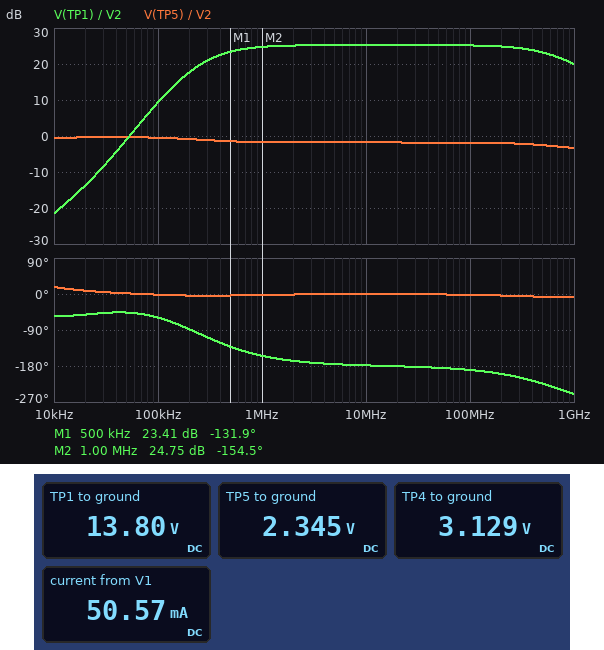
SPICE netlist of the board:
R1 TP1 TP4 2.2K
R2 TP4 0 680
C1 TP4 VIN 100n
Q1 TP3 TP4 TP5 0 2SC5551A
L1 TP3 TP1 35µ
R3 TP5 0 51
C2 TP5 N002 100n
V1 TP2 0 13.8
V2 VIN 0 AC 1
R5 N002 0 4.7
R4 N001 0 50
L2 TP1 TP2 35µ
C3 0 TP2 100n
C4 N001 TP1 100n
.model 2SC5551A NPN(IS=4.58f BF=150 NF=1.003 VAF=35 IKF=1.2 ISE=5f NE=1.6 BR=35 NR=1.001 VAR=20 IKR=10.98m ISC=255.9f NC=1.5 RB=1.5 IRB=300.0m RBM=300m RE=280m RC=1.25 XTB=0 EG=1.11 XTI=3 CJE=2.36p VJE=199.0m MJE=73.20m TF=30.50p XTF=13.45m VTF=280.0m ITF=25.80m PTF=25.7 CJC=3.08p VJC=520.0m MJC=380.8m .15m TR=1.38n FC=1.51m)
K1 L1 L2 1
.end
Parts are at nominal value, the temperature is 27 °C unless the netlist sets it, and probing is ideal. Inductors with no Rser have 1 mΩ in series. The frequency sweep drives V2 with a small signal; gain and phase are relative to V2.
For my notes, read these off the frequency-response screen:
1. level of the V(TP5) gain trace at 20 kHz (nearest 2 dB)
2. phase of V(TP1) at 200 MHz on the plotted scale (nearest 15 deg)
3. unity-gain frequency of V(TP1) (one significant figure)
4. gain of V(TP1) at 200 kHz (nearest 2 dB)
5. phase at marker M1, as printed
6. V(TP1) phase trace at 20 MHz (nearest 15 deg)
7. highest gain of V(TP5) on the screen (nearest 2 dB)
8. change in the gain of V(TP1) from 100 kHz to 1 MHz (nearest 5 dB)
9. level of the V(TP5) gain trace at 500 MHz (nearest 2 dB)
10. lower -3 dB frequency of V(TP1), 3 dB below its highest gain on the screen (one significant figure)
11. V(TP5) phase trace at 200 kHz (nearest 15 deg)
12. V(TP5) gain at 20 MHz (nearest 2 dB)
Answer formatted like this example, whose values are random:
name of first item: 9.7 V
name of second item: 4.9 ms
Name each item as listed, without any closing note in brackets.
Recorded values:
level of the V(TP5) gain trace at 20 kHz: 0 dB
phase of V(TP1) at 200 MHz on the plotted scale: -195 deg
unity-gain frequency of V(TP1): 50 kHz
gain of V(TP1) at 200 kHz: 18 dB
phase at marker M1, as printed: -131.9 deg
V(TP1) phase trace at 20 MHz: -180 deg
highest gain of V(TP5) on the screen: 0 dB
change in the gain of V(TP1) from 100 kHz to 1 MHz: 15 dB
level of the V(TP5) gain trace at 500 MHz: -2 dB
lower -3 dB frequency of V(TP1), 3 dB below its highest gain on the screen: 400 kHz
V(TP5) phase trace at 200 kHz: 0 deg
V(TP5) gain at 20 MHz: -2 dB
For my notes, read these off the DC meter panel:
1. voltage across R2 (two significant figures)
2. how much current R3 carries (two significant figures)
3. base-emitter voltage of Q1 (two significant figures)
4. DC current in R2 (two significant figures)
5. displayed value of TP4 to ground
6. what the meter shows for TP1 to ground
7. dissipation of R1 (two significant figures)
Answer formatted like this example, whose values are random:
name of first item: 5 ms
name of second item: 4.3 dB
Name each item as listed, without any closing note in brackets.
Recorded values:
voltage across R2: 3.1 V
how much current R3 carries: 46 mA
base-emitter voltage of Q1: 780 mV
DC current in R2: 4.6 mA
displayed value of TP4 to ground: 3.129 V
what the meter shows for TP1 to ground: 13.80 V
dissipation of R1: 52 mW
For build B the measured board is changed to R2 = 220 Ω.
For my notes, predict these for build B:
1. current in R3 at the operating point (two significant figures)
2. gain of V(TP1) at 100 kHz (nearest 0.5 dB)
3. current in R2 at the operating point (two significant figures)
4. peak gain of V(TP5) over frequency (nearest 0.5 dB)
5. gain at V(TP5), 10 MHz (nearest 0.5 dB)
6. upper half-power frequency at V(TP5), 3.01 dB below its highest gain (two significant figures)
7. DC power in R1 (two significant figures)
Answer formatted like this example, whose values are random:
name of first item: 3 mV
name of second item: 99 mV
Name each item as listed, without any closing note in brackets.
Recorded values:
current in R3 at the operating point: 10 mA
gain of V(TP1) at 100 kHz: 8.5 dB
current in R2 at the operating point: 5.7 mA
peak gain of V(TP5) over frequency: -1.0 dB
gain at V(TP5), 10 MHz: -4.5 dB
upper half-power frequency at V(TP5), 3.01 dB below its highest gain: 540 kHz
DC power in R1: 72 mW
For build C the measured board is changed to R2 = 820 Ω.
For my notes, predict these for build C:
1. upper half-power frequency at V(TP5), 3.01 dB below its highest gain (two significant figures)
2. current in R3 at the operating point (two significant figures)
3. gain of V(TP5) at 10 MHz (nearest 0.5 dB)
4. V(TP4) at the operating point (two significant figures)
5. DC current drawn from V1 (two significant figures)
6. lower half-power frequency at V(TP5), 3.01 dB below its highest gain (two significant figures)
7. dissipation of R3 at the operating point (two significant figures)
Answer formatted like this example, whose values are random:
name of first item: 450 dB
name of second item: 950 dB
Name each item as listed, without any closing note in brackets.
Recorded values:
upper half-power frequency at V(TP5), 3.01 dB below its highest gain: 1.1 GHz
current in R3 at the operating point: 54 mA
gain of V(TP5) at 10 MHz: -1.5 dB
V(TP4) at the operating point: 3.6 V
DC current drawn from V1: 59 mA
lower half-power frequency at V(TP5), 3.01 dB below its highest gain: 2.8 kHz
dissipation of R3 at the operating point: 150 mW
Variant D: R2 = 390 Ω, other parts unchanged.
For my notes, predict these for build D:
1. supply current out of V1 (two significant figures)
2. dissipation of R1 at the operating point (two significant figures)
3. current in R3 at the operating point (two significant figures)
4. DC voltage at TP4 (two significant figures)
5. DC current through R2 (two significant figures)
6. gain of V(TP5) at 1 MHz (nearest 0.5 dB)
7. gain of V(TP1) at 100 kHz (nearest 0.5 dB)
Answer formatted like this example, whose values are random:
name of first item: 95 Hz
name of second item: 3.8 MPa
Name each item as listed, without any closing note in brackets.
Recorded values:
supply current out of V1: 30 mA
dissipation of R1 at the operating point: 63 mW
current in R3 at the operating point: 25 mA
DC voltage at TP4: 2.0 V
DC current through R2: 5.2 mA
gain of V(TP5) at 1 MHz: -2.5 dB
gain of V(TP1) at 100 kHz: 9.0 dB
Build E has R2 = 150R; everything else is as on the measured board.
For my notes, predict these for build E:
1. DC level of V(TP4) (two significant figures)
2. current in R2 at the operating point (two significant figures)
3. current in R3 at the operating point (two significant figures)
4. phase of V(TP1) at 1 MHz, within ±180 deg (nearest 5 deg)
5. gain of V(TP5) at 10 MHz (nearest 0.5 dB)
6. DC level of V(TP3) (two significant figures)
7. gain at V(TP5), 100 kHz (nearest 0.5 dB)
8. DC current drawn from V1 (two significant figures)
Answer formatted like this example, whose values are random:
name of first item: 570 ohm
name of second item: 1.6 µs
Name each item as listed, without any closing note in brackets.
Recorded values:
DC level of V(TP4): 880 mV
current in R2 at the operating point: 5.9 mA
current in R3 at the operating point: 3.4 mA
phase of V(TP1) at 1 MHz, within ±180 deg: -160 deg
gain of V(TP5) at 10 MHz: -9.0 dB
DC level of V(TP3): 14 V
gain at V(TP5), 100 kHz: -3.0 dB
DC current drawn from V1: 9.3 mA
